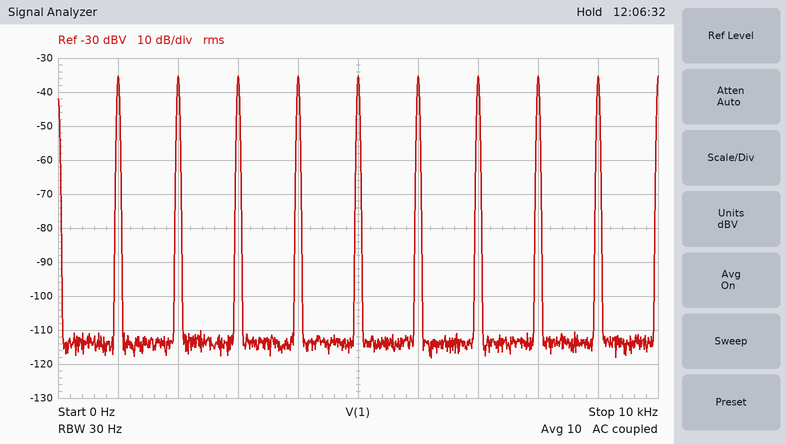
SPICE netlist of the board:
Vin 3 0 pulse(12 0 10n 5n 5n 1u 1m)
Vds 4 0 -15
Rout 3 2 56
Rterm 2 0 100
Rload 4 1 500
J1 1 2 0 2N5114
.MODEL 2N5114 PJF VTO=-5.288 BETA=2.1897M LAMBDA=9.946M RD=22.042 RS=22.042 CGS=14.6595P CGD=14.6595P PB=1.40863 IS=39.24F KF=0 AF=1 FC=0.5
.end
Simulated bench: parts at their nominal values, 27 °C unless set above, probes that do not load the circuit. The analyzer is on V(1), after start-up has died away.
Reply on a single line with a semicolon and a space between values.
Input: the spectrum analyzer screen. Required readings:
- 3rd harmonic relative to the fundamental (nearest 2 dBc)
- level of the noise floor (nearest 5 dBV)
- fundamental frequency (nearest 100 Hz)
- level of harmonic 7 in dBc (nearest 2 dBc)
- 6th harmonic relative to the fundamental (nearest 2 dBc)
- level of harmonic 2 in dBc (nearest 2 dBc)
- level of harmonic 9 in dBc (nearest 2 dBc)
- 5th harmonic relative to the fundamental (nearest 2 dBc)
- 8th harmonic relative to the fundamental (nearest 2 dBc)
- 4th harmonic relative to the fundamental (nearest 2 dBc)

0 dBc; -115 dBV; 1.0 kHz; 0 dBc; 0 dBc; 0 dBc; 0 dBc; 0 dBc; 0 dBc; 0 dBc
